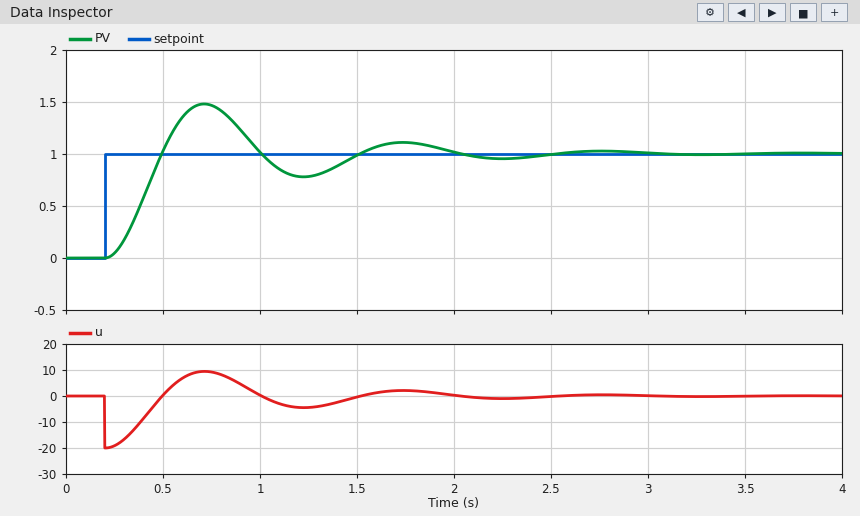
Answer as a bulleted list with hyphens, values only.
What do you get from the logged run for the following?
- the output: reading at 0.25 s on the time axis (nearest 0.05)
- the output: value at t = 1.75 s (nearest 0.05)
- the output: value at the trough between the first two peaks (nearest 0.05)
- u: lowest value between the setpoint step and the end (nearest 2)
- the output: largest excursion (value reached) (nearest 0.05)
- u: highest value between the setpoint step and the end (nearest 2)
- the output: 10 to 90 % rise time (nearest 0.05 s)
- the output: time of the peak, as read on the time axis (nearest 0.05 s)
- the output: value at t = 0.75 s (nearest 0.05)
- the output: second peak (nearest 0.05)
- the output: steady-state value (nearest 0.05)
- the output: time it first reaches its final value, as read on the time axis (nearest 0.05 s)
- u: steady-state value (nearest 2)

- 0.05
- 1.10
- 0.80
- -20
- 1.50
- 10
- 0.20 s
- 0.70 s
- 1.45
- 1.10
- 1.00
- 0.50 s
- 0
